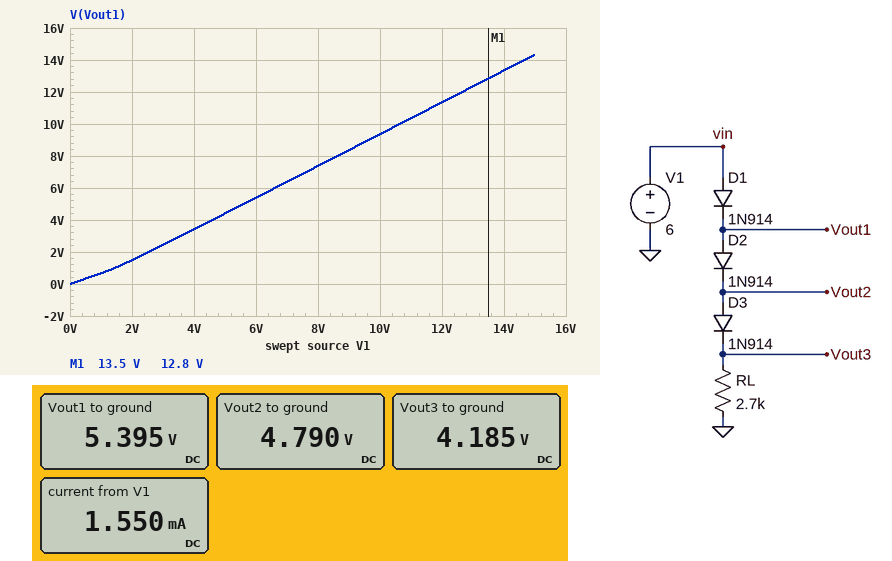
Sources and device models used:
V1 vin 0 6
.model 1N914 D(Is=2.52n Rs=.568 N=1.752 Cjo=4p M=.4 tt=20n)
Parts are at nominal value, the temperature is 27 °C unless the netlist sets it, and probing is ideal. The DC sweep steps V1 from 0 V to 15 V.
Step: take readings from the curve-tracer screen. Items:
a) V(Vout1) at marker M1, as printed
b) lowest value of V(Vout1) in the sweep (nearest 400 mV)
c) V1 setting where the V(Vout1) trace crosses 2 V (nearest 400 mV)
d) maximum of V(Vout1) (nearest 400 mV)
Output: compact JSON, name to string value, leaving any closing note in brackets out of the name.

{"V(Vout1) at marker M1, as printed": "12.8 V", "lowest value of V(Vout1) in the sweep": "0 V", "V1 setting where the V(Vout1) trace crosses 2 V": "2.4 V", "maximum of V(Vout1)": "14.4 V"}
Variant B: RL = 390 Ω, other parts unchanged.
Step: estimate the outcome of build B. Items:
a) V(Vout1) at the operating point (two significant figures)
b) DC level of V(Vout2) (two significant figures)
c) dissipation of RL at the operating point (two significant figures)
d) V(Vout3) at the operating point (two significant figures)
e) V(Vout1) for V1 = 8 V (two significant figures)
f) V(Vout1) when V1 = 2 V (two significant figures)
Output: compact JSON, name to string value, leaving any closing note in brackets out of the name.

{"V(Vout1) at the operating point": "5.3 V", "DC level of V(Vout2)": "4.6 V", "dissipation of RL at the operating point": "39 mW", "V(Vout3) at the operating point": "3.9 V", "V(Vout1) for V1 = 8 V": "7.3 V", "V(Vout1) when V1 = 2 V": "1.4 V"}
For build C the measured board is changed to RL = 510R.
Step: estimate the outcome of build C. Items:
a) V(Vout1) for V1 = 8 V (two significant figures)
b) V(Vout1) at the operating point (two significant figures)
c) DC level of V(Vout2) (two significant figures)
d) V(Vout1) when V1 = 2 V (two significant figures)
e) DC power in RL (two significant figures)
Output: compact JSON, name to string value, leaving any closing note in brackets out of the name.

{"V(Vout1) for V1 = 8 V": "7.3 V", "V(Vout1) at the operating point": "5.3 V", "DC level of V(Vout2)": "4.6 V", "V(Vout1) when V1 = 2 V": "1.4 V", "DC power in RL": "31 mW"}
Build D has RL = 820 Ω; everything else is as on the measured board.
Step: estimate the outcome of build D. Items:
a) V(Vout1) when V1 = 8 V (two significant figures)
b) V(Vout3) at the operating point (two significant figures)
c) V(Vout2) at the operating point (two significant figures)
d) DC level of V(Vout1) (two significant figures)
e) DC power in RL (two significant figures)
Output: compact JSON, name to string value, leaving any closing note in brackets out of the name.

{"V(Vout1) when V1 = 8 V": "7.3 V", "V(Vout3) at the operating point": "4.0 V", "V(Vout2) at the operating point": "4.7 V", "DC level of V(Vout1)": "5.3 V", "DC power in RL": "20 mW"}
